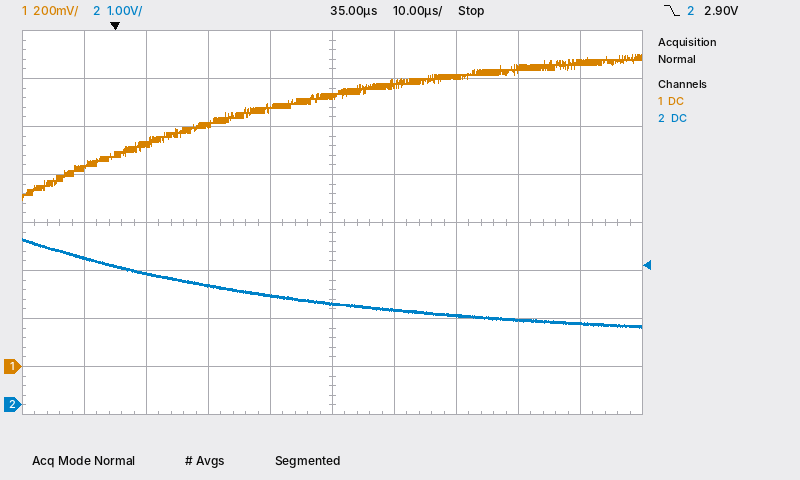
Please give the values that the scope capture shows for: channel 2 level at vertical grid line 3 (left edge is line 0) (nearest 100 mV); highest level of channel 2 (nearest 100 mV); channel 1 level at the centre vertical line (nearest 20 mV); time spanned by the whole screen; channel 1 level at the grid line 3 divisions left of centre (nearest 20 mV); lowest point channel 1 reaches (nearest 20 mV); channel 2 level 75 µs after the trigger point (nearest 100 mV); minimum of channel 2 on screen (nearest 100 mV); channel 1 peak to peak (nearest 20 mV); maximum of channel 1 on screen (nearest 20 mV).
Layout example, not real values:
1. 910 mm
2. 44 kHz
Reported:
1. 2.5 V
2. 3.5 V
3. 1.12 V
4. 100 µs
5. 920 mV
6. 700 mV
7. 1.7 V
8. 1.6 V
9. 600 mV
10. 1.30 V
